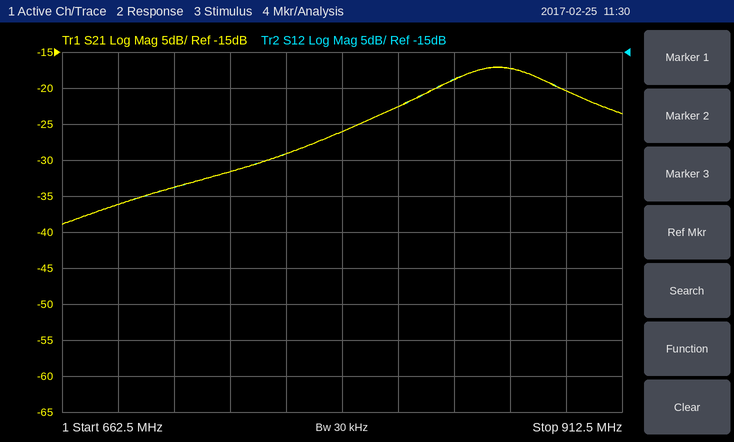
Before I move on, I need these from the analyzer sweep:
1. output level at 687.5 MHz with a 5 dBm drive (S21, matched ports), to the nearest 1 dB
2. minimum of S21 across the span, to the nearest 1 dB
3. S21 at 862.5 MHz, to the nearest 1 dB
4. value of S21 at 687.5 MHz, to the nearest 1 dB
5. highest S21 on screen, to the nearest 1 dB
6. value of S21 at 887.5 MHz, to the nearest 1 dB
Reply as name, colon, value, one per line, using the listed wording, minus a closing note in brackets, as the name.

output level at 687.5 MHz with a 5 dBm drive (S21, matched ports), to the nearest 1 dB: -31 dBm
minimum of S21 across the span, to the nearest 1 dB: -39 dB
S21 at 862.5 MHz, to the nearest 1 dB: -17 dB
value of S21 at 687.5 MHz, to the nearest 1 dB: -36 dB
highest S21 on screen, to the nearest 1 dB: -17 dB
value of S21 at 887.5 MHz, to the nearest 1 dB: -20 dB
